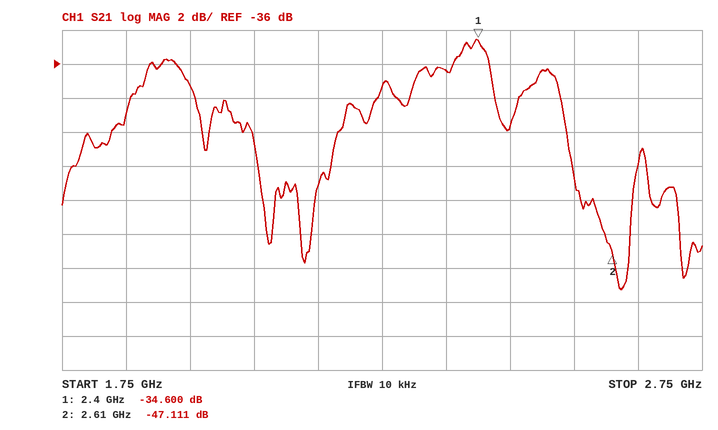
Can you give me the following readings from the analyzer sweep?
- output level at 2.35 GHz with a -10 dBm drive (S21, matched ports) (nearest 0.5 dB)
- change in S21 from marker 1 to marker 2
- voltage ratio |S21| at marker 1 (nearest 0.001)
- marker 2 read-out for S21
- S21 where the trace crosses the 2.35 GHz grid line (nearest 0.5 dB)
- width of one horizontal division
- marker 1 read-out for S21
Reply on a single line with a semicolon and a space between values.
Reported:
-46.5 dBm; -12.511 dB; 0.019; -47.111 dB; -36.5 dB; 100 MHz; -34.600 dB
